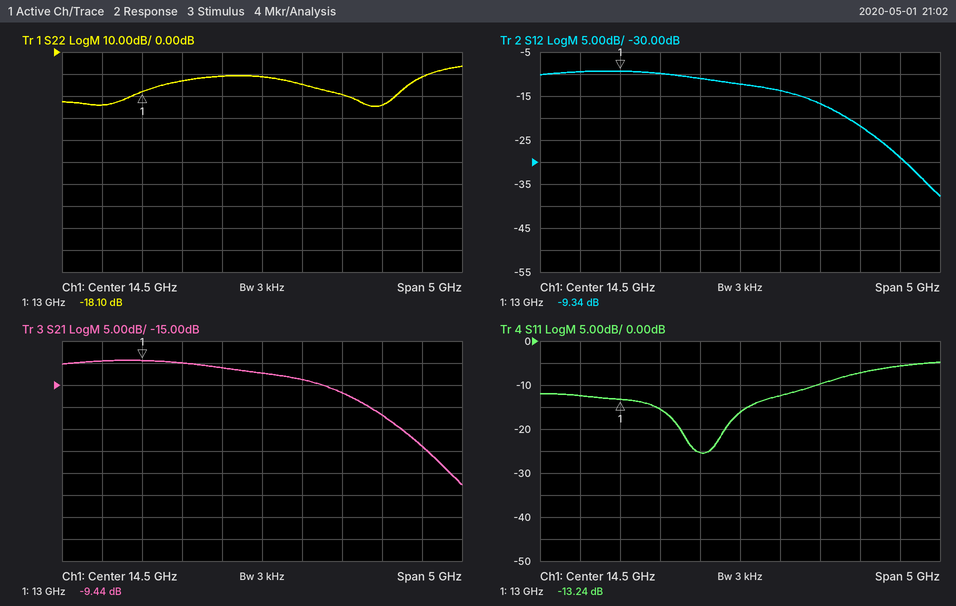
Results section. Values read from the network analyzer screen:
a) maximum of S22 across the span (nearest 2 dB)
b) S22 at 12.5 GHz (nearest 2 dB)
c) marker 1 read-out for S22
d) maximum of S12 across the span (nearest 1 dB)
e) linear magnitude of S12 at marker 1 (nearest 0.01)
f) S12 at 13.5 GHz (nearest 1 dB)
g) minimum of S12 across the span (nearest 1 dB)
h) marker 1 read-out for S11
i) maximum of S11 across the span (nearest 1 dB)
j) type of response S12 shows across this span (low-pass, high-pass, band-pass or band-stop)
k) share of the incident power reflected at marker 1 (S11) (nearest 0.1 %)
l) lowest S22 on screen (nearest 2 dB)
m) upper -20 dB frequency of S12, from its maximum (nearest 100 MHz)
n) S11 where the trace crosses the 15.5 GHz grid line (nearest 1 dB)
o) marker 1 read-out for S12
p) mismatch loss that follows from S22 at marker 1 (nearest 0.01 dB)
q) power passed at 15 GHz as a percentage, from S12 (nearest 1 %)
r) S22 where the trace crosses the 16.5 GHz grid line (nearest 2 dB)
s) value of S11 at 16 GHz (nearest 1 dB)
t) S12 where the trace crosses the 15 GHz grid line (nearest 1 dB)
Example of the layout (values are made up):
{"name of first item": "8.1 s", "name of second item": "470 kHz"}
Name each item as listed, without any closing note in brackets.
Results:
{"maximum of S22 across the span": "-6 dB", "S22 at 12.5 GHz": "-24 dB", "marker 1 read-out for S22": "-18.10 dB", "maximum of S12 across the span": "-9 dB", "linear magnitude of S12 at marker 1": "0.34", "S12 at 13.5 GHz": "-10 dB", "minimum of S12 across the span": "-38 dB", "marker 1 read-out for S11": "-13.24 dB", "maximum of S11 across the span": "-5 dB", "type of response S12 shows across this span": "low-pass", "share of the incident power reflected at marker 1 (S11)": "4.7 %", "lowest S22 on screen": "-24 dB", "upper -20 dB frequency of S12, from its maximum": "16.5 GHz", "S11 where the trace crosses the 15.5 GHz grid line": "-10 dB", "marker 1 read-out for S12": "-9.34 dB", "mismatch loss that follows from S22 at marker 1": "0.07 dB", "power passed at 15 GHz as a percentage, from S12": "4 %", "S22 where the trace crosses the 16.5 GHz grid line": "-12 dB", "value of S11 at 16 GHz": "-7 dB", "S12 where the trace crosses the 15 GHz grid line": "-14 dB"}
